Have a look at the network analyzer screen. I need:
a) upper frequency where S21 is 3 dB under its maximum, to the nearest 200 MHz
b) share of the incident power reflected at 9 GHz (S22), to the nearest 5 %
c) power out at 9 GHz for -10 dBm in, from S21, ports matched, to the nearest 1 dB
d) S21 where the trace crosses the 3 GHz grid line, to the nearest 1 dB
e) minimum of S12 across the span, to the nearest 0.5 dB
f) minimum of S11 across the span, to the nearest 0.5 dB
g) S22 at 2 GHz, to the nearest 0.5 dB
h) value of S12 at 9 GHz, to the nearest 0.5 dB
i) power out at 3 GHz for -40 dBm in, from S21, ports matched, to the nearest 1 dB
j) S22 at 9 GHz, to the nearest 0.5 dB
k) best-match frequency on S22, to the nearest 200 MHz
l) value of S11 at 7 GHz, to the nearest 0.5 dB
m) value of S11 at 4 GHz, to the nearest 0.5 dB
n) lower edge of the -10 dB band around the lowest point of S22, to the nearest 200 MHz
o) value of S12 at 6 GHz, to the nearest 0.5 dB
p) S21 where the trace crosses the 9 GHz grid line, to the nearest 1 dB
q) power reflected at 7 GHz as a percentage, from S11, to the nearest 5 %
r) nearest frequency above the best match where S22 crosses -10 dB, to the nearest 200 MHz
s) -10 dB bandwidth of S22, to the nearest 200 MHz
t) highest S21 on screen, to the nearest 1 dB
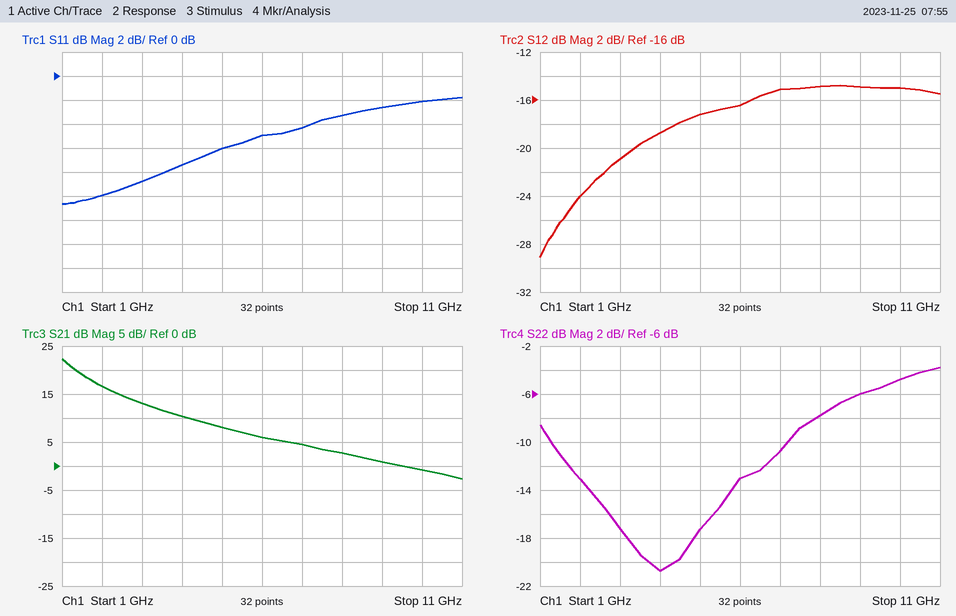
1.4 GHz
25 %
-9 dBm
13 dB
-29.0 dB
-10.5 dB
-13.0 dB
-15.0 dB
-27 dBm
-6.0 dB
4.0 GHz
-4.5 dB
-7.5 dB
1.2 GHz
-16.5 dB
1 dB
35 %
7.2 GHz
6.0 GHz
22 dB
